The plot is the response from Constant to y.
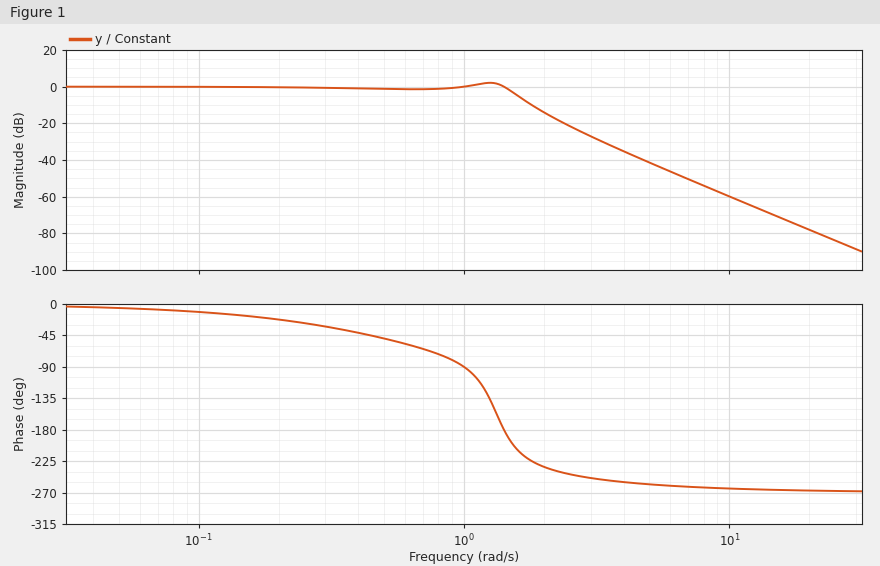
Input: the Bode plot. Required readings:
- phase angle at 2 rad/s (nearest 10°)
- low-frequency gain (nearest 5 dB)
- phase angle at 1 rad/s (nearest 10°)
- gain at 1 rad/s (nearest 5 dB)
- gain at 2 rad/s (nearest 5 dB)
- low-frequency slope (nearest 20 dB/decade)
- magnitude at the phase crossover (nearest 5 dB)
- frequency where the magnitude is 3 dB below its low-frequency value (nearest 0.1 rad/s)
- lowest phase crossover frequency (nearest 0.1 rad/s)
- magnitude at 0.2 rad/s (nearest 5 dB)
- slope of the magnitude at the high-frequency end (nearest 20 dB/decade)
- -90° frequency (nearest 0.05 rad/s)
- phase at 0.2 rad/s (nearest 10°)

-230°
0 dB
-90°
0 dB
-15 dB
0 dB/decade
0 dB
1.5 rad/s
1.4 rad/s
0 dB
-60 dB/decade
1.00 rad/s
-20°
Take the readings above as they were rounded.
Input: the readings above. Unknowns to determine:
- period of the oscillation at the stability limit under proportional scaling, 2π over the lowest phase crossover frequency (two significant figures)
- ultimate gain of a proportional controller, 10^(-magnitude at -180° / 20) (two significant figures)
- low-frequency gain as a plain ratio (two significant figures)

4.5 s
1.0
1.0
